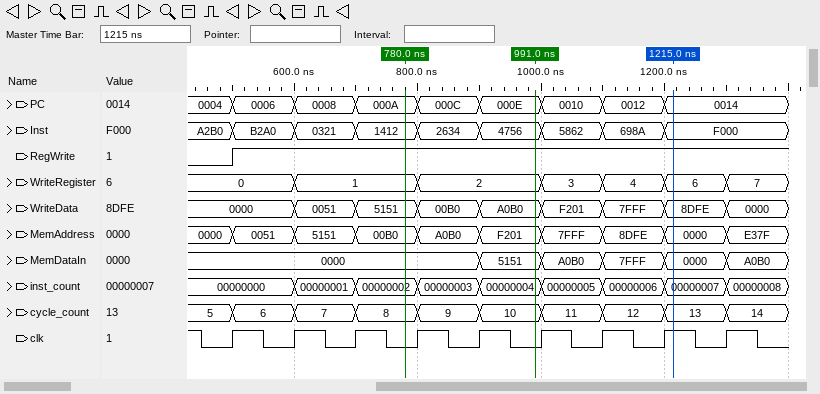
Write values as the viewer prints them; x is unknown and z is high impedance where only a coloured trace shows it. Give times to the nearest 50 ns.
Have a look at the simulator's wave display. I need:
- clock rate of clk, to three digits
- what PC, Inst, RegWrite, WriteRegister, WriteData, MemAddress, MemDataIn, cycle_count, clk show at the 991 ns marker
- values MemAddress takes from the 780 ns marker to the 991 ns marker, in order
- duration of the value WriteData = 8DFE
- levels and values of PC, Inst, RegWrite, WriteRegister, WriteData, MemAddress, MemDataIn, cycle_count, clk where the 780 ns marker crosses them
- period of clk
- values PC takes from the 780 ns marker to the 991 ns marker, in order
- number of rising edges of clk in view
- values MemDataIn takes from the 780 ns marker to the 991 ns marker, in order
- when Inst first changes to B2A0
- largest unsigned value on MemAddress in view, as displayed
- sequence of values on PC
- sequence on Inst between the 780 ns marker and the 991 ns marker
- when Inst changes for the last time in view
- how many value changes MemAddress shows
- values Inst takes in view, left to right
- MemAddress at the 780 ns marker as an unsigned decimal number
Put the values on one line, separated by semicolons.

10.0 MHz; PC=000E, Inst=4756, RegWrite=1, WriteRegister=2, WriteData=A0B0, MemAddress=F201, MemDataIn=5151, cycle_count=10, clk=0; 00B0, A0B0, F201; 100 ns; PC=000A, Inst=1412, RegWrite=1, WriteRegister=1, WriteData=5151, MemAddress=00B0, MemDataIn=0000, cycle_count=8, clk=0; 100 ns; 000A, 000C, 000E; 9; 0000, 5151; 500 ns; F201; 0004, 0006, 0008, 000A, 000C, 000E, 0010, 0012, 0014; 1412, 2634, 4756; 1200 ns; 9; A2B0, B2A0, 0321, 1412, 2634, 4756, 5862, 698A, F000; 176
